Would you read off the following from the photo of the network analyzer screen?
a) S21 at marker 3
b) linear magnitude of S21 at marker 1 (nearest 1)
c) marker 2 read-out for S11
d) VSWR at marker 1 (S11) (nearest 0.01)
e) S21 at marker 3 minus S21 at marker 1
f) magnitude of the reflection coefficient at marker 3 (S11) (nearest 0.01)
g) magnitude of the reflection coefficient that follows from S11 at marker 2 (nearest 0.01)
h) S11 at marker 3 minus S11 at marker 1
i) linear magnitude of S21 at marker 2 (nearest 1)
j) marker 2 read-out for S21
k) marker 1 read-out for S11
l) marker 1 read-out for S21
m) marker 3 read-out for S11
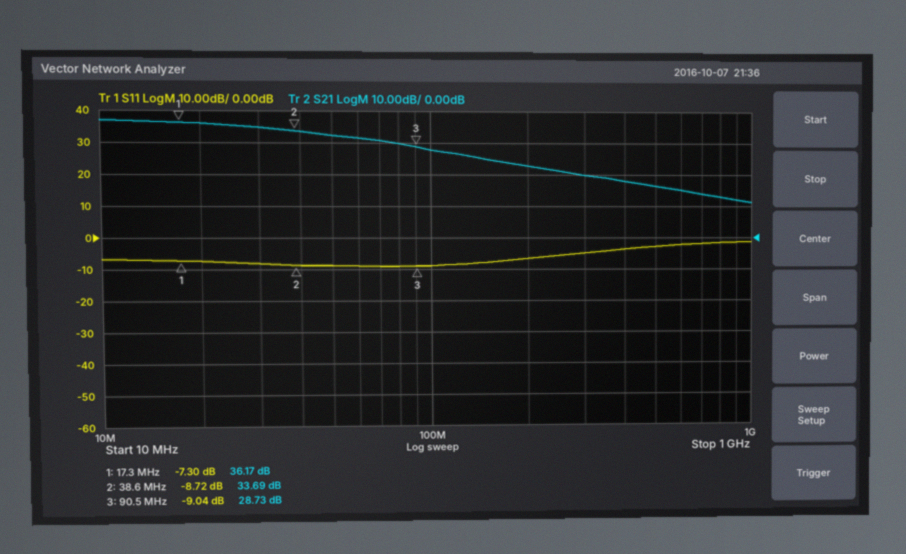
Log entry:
28.73 dB
64
-8.72 dB
2.52
-7.44 dB
0.35
0.37
-1.74 dB
48
33.69 dB
-7.30 dB
36.17 dB
-9.04 dB
